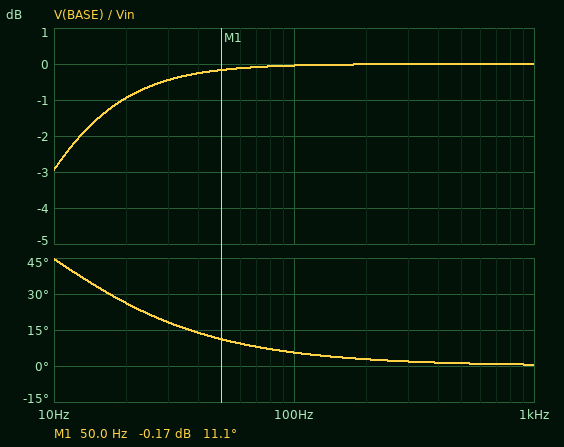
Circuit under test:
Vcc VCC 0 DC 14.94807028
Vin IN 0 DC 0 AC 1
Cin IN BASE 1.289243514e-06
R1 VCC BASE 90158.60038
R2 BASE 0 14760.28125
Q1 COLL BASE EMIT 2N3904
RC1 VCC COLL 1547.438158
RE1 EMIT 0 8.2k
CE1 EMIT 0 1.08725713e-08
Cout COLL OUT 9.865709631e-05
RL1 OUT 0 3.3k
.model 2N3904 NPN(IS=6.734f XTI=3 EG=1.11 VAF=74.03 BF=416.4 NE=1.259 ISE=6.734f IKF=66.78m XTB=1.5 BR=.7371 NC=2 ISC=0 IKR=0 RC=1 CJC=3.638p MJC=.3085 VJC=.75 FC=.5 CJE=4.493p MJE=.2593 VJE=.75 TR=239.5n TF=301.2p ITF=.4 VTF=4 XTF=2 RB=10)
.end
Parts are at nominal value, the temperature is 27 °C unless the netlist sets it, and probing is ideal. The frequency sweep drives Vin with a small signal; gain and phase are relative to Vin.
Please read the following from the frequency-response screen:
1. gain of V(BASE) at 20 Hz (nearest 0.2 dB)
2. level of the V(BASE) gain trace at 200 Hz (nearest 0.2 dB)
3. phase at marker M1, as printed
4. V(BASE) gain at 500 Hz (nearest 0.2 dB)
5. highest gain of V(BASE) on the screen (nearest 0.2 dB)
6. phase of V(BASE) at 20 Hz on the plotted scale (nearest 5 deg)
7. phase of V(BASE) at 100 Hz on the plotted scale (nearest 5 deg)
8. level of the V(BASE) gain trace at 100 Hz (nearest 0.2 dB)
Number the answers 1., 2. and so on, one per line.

1. -1.0 dB
2. 0 dB
3. 11.1 deg
4. 0 dB
5. 0 dB
6. 25 deg
7. 5 deg
8. 0 dB
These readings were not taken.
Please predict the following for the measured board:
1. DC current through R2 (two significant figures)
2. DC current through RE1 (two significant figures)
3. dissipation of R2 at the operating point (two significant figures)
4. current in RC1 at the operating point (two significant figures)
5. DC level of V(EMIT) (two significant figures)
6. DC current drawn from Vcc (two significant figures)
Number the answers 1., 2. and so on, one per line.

1. 140 µA
2. 180 µA
3. 290 µW
4. 180 µA
5. 1.5 V
6. 320 µA
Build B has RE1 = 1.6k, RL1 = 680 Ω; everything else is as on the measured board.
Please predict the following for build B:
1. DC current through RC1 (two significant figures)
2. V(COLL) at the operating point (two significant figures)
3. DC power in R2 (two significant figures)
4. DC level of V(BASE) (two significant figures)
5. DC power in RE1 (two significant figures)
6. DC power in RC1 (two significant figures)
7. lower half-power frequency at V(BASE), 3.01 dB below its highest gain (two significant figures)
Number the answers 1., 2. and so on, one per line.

1. 850 µA
2. 14 V
3. 280 µW
4. 2.0 V
5. 1.2 mW
6. 1.1 mW
7. 10 Hz
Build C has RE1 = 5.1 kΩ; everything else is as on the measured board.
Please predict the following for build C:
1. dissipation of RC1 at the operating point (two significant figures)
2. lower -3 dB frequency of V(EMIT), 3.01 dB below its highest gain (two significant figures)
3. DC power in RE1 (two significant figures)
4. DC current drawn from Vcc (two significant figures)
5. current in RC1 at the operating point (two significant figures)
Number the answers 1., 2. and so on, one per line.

1. 120 µW
2. 9.9 Hz
3. 410 µW
4. 420 µA
5. 280 µA
